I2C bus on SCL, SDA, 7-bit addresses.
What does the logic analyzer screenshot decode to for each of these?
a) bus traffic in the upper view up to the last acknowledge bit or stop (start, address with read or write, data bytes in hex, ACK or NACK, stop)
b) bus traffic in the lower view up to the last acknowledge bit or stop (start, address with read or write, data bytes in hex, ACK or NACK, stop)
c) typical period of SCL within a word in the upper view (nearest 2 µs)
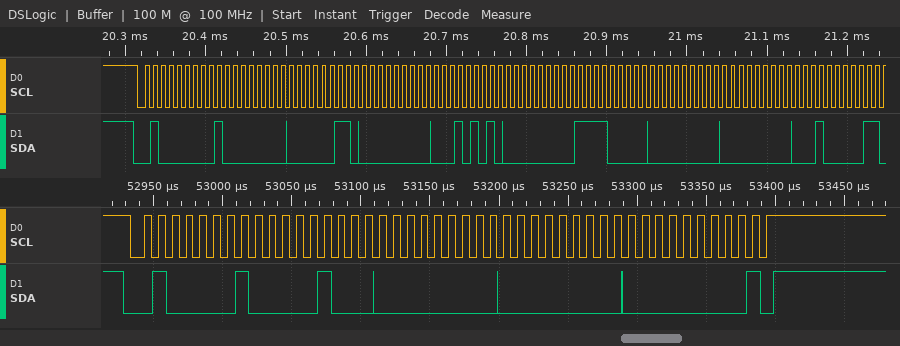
start, address 20 write ACK, 80 ACK, 03 ACK, 00 ACK, 15 ACK, 00 ACK, F0 ACK, 00 ACK, 00 ACK, 10 ACK
start, address 20 read ACK, 08 ACK, 00 ACK, 00 ACK, 00 NACK, stop
10 µs
